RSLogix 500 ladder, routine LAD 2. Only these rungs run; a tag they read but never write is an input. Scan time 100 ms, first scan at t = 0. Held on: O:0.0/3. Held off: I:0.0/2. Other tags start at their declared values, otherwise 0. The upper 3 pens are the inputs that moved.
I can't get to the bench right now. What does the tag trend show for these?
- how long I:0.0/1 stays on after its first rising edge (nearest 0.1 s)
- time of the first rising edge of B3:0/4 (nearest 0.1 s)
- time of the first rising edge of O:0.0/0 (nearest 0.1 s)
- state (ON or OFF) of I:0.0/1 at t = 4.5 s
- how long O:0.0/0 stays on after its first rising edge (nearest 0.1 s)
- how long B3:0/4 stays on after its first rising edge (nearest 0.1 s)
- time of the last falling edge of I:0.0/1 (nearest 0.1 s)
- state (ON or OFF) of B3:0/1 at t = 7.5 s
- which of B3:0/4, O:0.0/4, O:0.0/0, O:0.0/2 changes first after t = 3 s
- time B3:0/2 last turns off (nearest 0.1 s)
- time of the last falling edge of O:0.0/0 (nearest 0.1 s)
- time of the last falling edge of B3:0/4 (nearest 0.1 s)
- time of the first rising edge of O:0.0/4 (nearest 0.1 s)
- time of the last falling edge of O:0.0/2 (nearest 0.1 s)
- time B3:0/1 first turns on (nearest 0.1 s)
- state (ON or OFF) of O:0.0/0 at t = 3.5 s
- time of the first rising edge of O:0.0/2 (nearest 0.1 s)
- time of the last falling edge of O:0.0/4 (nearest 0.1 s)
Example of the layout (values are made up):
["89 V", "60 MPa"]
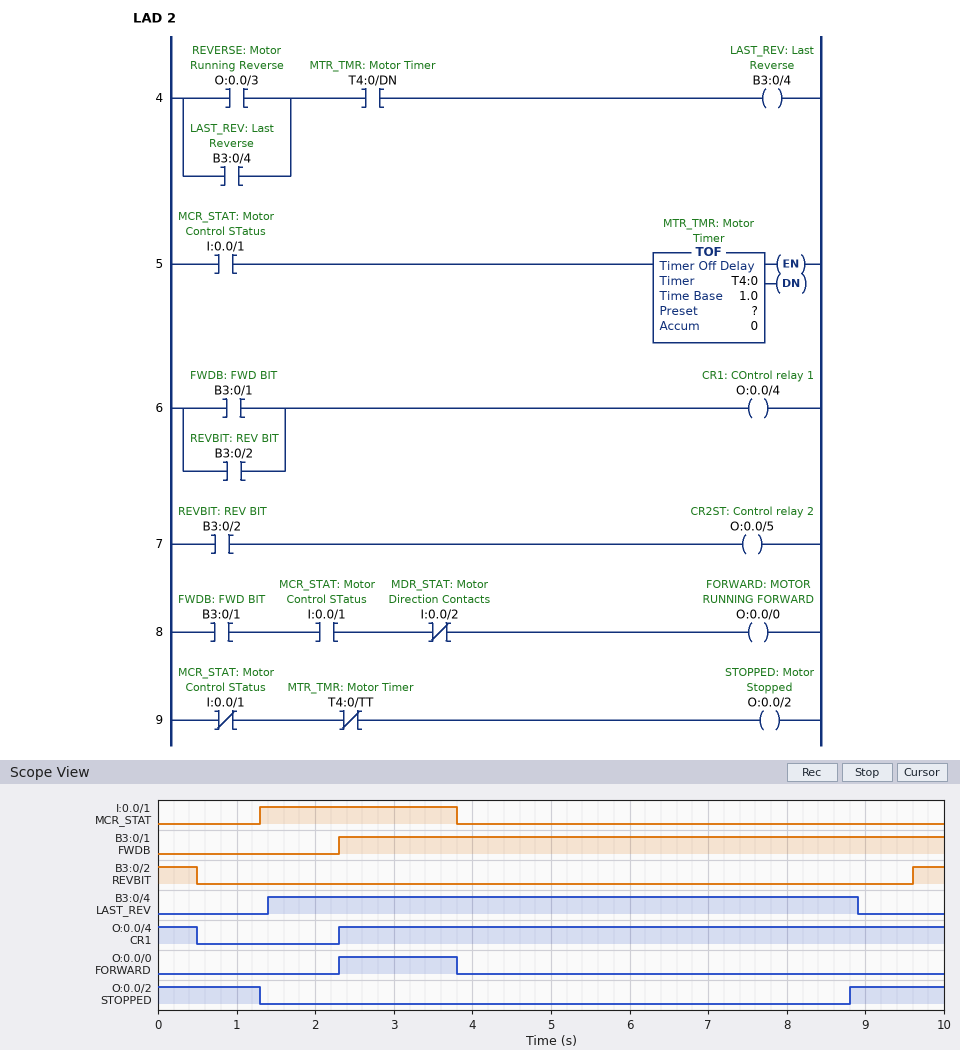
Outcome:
["2.5 s", "1.4 s", "2.3 s", "OFF", "1.5 s", "7.5 s", "3.8 s", "ON", "O:0.0/0", "0.5 s", "3.8 s", "8.9 s", "2.3 s", "1.3 s", "2.3 s", "ON", "8.8 s", "0.5 s"]
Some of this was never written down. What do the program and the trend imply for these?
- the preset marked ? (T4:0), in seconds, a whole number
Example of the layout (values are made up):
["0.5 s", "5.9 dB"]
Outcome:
["5 s"]
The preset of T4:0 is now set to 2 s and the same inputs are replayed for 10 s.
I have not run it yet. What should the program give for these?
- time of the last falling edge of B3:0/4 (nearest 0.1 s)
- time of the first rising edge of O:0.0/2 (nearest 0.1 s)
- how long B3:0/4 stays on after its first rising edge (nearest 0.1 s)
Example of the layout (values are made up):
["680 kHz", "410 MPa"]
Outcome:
["5.9 s", "5.8 s", "4.5 s"]
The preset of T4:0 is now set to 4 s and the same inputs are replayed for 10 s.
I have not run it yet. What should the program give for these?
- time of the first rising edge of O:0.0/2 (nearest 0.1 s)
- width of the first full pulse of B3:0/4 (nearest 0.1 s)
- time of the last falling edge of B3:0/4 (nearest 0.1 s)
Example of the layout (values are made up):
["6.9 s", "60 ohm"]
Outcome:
["7.8 s", "6.5 s", "7.9 s"]
